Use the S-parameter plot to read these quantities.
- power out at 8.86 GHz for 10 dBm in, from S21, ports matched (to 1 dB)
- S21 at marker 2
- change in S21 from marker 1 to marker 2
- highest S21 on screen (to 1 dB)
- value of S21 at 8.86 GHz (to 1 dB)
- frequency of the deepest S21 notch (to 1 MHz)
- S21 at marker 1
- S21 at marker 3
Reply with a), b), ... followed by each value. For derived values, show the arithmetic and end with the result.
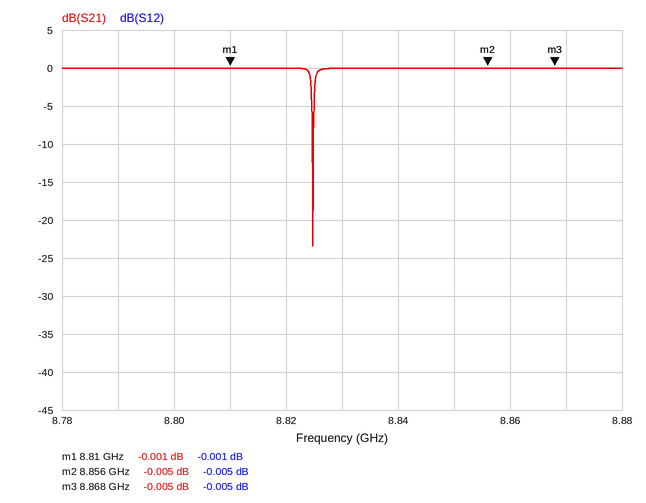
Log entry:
a) 10 dBm + (0 dB) = 10 dBm
b) -0.005 dB
c) -0.005 − (-0.001) = -0.004 dB
d) 0 dB
e) 0 dB
f) 8.825 GHz
g) -0.001 dB
h) -0.005 dB
